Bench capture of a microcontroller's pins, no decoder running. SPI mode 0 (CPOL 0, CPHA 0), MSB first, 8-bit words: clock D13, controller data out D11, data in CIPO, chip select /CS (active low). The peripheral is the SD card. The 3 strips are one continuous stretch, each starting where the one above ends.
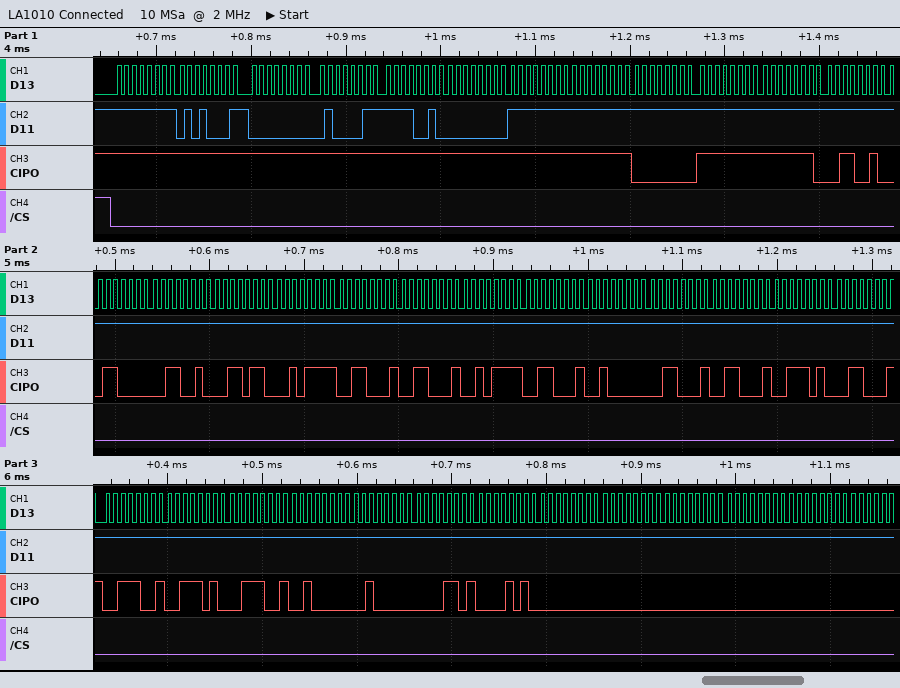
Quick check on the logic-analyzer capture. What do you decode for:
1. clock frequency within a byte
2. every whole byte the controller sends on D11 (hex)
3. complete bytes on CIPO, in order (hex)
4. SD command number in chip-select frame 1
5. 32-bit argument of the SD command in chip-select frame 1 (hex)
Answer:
125 kHz
FF 51 00 43 F2 00 FF FF FF FF FF FF FF FF FF FF FF FF FF FF FF FF FF FF FF FF FF FF FF FF FF FF FF FF FF FF FF
FF FF FF FF FF FF FF FF 00 FF FE 32 30 32 36 2F 31 31 2F 31 20 31 31 3A 31 39 3A 39 20 20 0D 0A 00 00 00 00 00
CMD17
0x0043F200
